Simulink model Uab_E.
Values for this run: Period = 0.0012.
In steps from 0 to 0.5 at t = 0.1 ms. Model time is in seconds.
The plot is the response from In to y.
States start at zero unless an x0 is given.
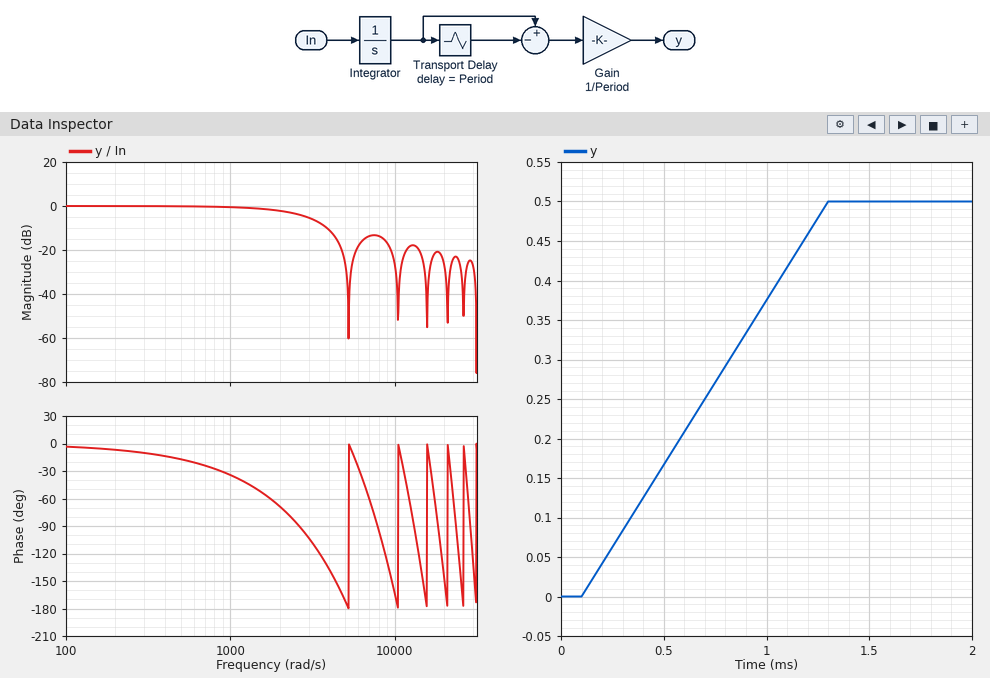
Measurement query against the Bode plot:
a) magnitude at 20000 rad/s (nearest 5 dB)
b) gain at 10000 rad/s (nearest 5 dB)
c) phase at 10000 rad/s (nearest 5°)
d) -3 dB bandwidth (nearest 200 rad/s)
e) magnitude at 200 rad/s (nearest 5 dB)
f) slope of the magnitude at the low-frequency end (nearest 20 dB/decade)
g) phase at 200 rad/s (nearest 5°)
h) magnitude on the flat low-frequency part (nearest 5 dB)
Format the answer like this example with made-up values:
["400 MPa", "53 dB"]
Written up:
["-25 dB", "-25 dB", "-165°", "2400 rad/s", "0 dB", "0 dB/decade", "-5°", "0 dB"]
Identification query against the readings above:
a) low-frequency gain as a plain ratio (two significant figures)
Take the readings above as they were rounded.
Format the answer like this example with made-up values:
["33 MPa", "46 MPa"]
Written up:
["1.0"]
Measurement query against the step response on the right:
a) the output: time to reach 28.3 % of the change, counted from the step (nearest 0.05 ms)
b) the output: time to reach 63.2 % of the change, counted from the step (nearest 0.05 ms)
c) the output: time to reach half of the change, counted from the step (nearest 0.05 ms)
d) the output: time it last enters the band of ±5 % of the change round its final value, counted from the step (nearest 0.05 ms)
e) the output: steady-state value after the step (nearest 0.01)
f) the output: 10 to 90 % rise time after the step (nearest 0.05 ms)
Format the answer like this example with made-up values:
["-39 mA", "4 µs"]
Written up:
["0.35 ms", "0.75 ms", "0.60 ms", "1.15 ms", "0.50", "0.95 ms"]
